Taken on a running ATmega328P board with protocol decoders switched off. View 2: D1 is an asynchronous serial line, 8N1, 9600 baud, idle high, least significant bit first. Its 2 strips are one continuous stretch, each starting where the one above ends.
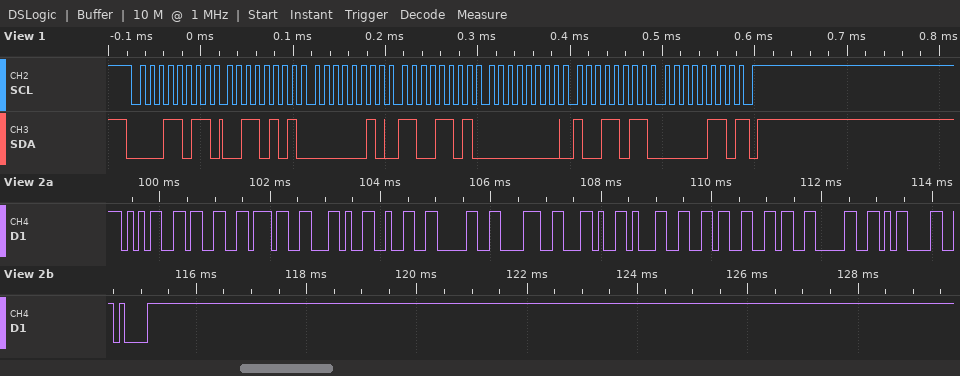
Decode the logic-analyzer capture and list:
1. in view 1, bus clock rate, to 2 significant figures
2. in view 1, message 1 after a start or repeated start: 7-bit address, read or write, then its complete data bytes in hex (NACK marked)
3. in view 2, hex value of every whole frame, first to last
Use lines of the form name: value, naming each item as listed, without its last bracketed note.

in view 1, bus clock rate, to 2 significant figures: 100 kHz
in view 1, message 1 after a start or repeated start: 7-bit address, read or write, then its complete data bytes in hex: 0x0D read: 35 02 CD 00 9B 06 NACK
in view 2, hex value of every whole frame, first to last: 35 33 37 2C 32 30 38 2C 31 36 36 30 0D 0A
